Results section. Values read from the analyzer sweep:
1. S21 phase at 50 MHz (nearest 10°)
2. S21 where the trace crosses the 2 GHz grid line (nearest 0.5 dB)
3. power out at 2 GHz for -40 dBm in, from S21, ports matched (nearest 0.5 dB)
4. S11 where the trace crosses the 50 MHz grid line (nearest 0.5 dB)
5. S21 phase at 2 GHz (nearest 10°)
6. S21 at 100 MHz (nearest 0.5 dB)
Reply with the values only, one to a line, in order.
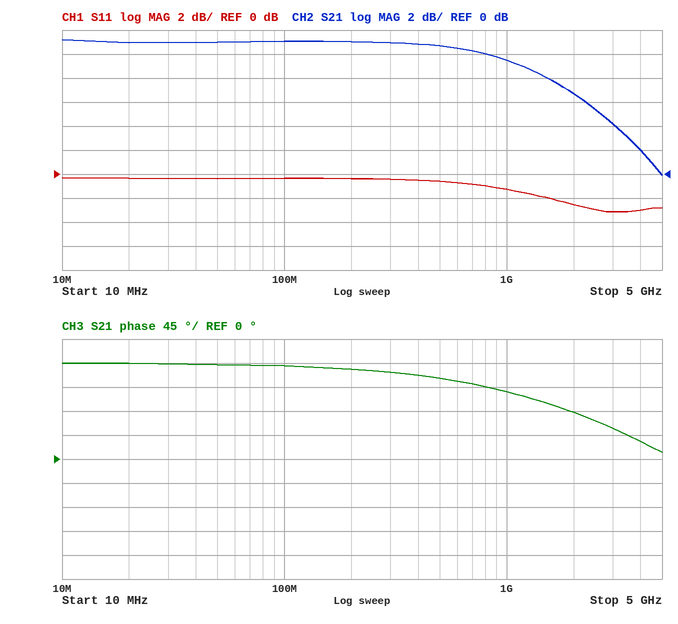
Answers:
180°
6.5 dB
-33.5 dBm
-0.5 dB
90°
11.0 dB
